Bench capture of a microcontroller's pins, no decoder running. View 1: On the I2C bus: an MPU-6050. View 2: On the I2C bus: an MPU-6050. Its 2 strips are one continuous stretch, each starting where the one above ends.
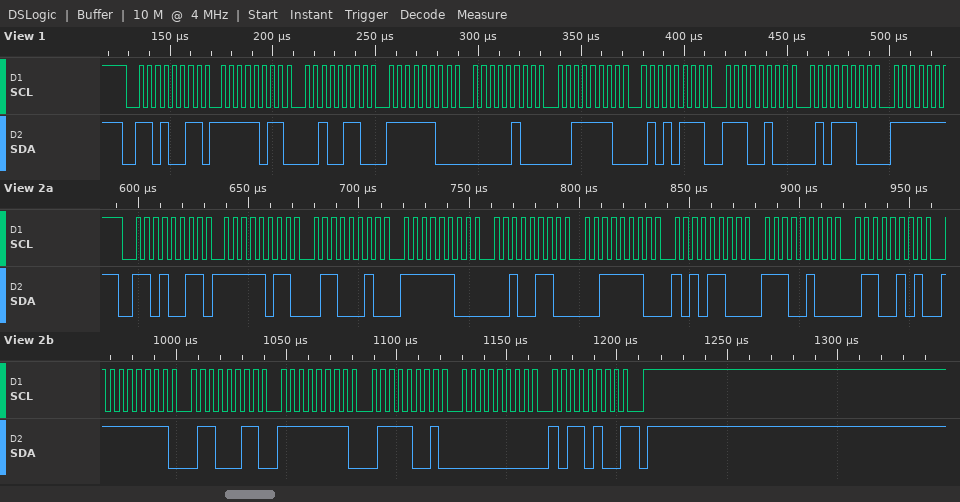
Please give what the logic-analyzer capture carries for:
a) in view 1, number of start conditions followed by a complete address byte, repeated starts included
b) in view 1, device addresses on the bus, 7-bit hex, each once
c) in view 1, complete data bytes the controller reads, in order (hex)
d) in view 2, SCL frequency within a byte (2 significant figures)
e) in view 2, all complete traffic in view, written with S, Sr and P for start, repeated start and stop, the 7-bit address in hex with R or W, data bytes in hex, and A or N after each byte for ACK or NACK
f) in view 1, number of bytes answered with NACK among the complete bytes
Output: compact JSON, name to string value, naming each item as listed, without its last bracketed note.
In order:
{"in view 1, number of start conditions followed by a complete address byte, repeated starts included": "1", "in view 1, device addresses on the bus, 7-bit hex, each once": "0x69", "in view 1, complete data bytes the controller reads, in order": "FB 26 FC 04 3E 57 E4 5C", "in view 2, SCL frequency within a byte": "250 kHz", "in view 2, all complete traffic in view, written with S, Sr and P for start, repeated start and stop, the 7-bit address in hex with R or W, data bytes in hex, and A or N after each byte for ACK or NACK": "S 69R A FB A 62 A FC A 26 A 3E A AC A E4 A 65 A FF A 63 A FF A 79 A 00 A B4 N P", "in view 1, number of bytes answered with NACK among the complete bytes": "0"}
